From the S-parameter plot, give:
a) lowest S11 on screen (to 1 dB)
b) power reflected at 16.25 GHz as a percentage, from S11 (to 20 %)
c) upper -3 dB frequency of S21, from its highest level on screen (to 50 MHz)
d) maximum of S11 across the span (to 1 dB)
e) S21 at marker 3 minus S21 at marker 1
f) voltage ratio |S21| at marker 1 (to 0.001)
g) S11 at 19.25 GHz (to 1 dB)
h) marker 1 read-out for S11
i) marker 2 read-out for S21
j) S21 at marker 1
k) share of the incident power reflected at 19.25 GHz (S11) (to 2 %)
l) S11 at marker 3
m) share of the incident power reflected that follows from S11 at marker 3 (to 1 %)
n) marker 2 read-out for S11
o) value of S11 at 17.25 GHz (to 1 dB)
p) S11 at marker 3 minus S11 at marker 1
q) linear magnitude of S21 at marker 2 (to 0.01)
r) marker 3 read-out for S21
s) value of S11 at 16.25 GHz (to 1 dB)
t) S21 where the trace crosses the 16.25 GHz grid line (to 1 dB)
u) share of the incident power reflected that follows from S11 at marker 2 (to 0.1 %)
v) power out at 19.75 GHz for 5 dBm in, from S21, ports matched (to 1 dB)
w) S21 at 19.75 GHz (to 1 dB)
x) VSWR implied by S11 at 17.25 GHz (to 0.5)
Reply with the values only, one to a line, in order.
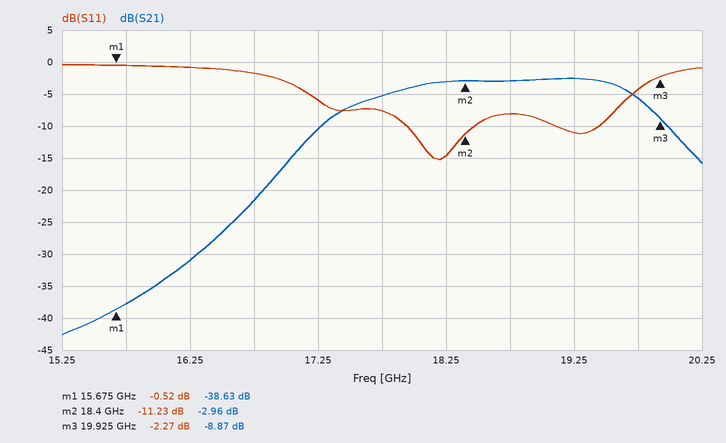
-15 dB
80 %
19.75 GHz
0 dB
29.76 dB
0.012
-11 dB
-0.52 dB
-2.96 dB
-38.63 dB
8 %
-2.27 dB
59 %
-11.23 dB
-6 dB
-1.75 dB
0.71
-8.87 dB
-1 dB
-31 dB
7.5 %
-1 dBm
-6 dB
3.0
